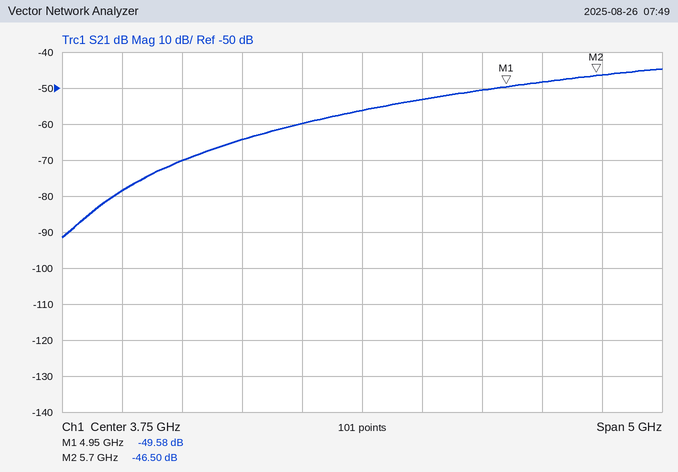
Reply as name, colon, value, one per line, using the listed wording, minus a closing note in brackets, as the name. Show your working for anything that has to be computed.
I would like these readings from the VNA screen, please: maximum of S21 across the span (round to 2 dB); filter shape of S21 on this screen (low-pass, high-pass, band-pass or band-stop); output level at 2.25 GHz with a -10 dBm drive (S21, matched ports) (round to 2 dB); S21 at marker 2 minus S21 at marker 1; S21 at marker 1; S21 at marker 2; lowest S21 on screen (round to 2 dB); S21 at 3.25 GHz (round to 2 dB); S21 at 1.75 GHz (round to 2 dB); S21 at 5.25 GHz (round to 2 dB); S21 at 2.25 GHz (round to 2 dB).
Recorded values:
maximum of S21 across the span: -44 dB
filter shape of S21 on this screen: high-pass
output level at 2.25 GHz with a -10 dBm drive (S21, matched ports): -10 dBm + (-70 dB) = -80 dBm
S21 at marker 2 minus S21 at marker 1: -46.5 − (-49.58) = 3.08 dB
S21 at marker 1: -49.58 dB
S21 at marker 2: -46.50 dB
lowest S21 on screen: -92 dB
S21 at 3.25 GHz: -60 dB
S21 at 1.75 GHz: -78 dB
S21 at 5.25 GHz: -48 dB
S21 at 2.25 GHz: -70 dB
